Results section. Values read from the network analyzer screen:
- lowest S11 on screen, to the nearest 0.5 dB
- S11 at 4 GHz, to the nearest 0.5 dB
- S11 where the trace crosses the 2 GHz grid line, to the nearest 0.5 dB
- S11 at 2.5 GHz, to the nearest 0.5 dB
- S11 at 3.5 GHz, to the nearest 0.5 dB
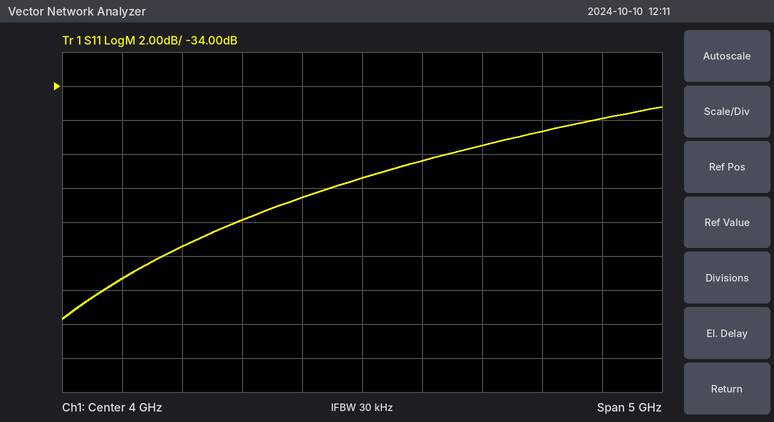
-47.5 dB
-39.5 dB
-45.5 dB
-43.5 dB
-40.5 dB
